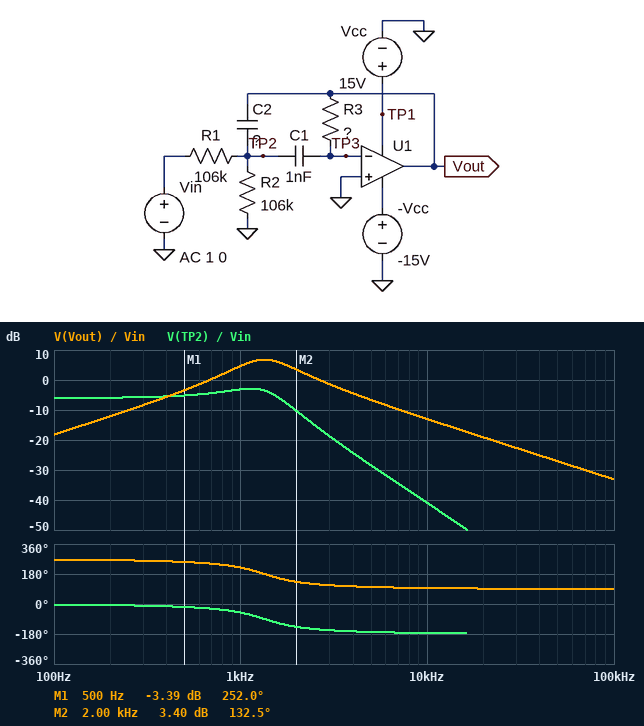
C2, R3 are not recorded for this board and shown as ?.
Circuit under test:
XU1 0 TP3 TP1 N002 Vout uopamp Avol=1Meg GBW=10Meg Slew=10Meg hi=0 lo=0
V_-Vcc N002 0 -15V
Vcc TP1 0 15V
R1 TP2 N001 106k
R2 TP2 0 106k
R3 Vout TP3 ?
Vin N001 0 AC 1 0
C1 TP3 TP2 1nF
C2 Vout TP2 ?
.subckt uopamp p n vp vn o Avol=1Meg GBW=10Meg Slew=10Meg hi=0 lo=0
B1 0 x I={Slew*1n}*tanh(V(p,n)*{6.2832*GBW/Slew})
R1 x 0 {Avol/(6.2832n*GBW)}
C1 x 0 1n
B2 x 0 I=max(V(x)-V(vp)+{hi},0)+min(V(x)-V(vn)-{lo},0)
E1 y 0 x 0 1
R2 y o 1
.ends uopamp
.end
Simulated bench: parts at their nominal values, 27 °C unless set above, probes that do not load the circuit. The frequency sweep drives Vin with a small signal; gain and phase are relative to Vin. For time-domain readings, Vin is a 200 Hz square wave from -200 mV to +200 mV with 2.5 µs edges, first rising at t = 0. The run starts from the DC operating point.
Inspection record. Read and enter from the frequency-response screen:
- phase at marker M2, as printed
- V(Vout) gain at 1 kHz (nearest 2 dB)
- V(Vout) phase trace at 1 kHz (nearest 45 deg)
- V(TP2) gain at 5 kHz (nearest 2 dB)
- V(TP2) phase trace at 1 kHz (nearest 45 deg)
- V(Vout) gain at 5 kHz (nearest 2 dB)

132.5 deg
4 dB
225 deg
-28 dB
-45 deg
-6 dB
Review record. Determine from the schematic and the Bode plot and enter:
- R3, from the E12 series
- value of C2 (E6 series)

390 kΩ
680 pF
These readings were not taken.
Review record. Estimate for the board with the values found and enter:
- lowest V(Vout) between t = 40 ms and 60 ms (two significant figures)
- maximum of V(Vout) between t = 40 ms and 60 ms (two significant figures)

-410 mV
410 mV
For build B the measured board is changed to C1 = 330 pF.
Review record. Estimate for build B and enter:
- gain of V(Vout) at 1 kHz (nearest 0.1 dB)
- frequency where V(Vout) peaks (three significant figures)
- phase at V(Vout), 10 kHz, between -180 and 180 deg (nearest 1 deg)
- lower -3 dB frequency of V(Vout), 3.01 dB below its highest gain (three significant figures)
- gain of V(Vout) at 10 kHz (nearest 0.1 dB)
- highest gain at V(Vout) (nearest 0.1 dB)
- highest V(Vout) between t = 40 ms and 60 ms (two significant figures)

-6.8 dB
2.34 kHz
101 deg
1.59 kHz
-12.8 dB
1.6 dB
230 mV
